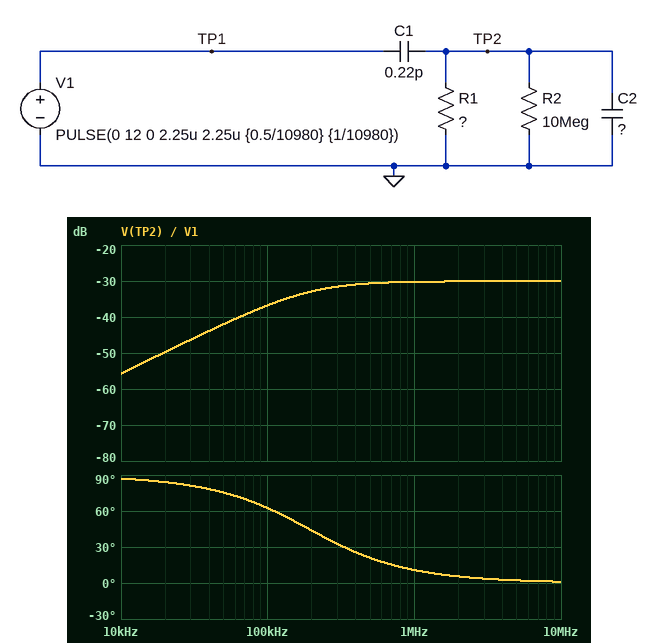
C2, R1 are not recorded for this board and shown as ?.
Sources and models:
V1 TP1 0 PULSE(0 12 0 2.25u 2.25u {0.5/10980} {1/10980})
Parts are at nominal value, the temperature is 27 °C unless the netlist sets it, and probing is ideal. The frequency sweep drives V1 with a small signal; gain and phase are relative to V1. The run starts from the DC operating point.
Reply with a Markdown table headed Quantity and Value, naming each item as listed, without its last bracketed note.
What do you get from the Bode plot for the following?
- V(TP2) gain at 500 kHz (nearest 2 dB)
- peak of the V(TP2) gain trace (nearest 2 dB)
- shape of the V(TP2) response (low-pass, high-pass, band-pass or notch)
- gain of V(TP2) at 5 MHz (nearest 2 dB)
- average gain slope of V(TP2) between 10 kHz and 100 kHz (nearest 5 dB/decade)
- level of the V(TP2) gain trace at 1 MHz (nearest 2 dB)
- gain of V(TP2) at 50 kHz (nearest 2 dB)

| Quantity | Value |
|---|---|
| V(TP2) gain at 500 kHz | -30 dB |
| peak of the V(TP2) gain trace | -30 dB |
| shape of the V(TP2) response | high-pass |
| gain of V(TP2) at 5 MHz | -30 dB |
| average gain slope of V(TP2) between 10 kHz and 100 kHz | 20 dB/decade |
| level of the V(TP2) gain trace at 1 MHz | -30 dB |
| gain of V(TP2) at 50 kHz | -42 dB |
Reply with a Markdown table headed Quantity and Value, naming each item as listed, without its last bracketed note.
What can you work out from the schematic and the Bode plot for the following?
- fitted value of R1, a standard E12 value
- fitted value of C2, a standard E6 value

| Quantity | Value |
|---|---|
| fitted value of R1, a standard E12 value | 120 kΩ |
| fitted value of C2, a standard E6 value | 6.8 pF |
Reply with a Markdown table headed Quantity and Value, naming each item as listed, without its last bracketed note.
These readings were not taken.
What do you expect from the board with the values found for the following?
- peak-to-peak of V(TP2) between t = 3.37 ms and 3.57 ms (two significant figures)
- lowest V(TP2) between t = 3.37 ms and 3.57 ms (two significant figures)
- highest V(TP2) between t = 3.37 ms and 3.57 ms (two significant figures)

| Quantity | Value |
|---|---|
| peak-to-peak of V(TP2) between t = 3.37 ms and 3.57 ms | 260 mV |
| lowest V(TP2) between t = 3.37 ms and 3.57 ms | -130 mV |
| highest V(TP2) between t = 3.37 ms and 3.57 ms | 130 mV |
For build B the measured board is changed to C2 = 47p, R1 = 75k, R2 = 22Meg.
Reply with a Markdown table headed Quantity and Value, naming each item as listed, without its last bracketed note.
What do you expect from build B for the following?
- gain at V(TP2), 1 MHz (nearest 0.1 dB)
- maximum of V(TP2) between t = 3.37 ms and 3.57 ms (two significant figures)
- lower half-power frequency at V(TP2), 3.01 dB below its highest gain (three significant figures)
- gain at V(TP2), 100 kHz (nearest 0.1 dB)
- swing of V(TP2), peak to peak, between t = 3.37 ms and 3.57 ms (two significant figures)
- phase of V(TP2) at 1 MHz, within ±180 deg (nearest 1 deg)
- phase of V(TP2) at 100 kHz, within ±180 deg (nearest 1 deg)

| Quantity | Value |
|---|---|
| gain at V(TP2), 1 MHz | -46.6 dB |
| maximum of V(TP2) between t = 3.37 ms and 3.57 ms | 41 mV |
| lower half-power frequency at V(TP2), 3.01 dB below its highest gain | 45.1 kHz |
| gain at V(TP2), 100 kHz | -47.4 dB |
| swing of V(TP2), peak to peak, between t = 3.37 ms and 3.57 ms | 83 mV |
| phase of V(TP2) at 1 MHz, within ±180 deg | 3 deg |
| phase of V(TP2) at 100 kHz, within ±180 deg | 24 deg |
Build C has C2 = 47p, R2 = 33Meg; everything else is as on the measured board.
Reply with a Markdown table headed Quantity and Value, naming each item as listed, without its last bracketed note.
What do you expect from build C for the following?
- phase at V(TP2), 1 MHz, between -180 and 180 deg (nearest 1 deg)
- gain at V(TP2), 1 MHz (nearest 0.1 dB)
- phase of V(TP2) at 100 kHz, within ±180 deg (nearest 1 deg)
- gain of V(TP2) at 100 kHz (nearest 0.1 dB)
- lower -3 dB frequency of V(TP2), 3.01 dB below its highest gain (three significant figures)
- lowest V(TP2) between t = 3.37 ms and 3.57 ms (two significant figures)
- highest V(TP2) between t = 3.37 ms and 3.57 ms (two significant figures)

| Quantity | Value |
|---|---|
| phase at V(TP2), 1 MHz, between -180 and 180 deg | 2 deg |
| gain at V(TP2), 1 MHz | -46.6 dB |
| phase of V(TP2) at 100 kHz, within ±180 deg | 16 deg |
| gain of V(TP2) at 100 kHz | -47.0 dB |
| lower -3 dB frequency of V(TP2), 3.01 dB below its highest gain | 28.2 kHz |
| lowest V(TP2) between t = 3.37 ms and 3.57 ms | -46 mV |
| highest V(TP2) between t = 3.37 ms and 3.57 ms | 46 mV |
